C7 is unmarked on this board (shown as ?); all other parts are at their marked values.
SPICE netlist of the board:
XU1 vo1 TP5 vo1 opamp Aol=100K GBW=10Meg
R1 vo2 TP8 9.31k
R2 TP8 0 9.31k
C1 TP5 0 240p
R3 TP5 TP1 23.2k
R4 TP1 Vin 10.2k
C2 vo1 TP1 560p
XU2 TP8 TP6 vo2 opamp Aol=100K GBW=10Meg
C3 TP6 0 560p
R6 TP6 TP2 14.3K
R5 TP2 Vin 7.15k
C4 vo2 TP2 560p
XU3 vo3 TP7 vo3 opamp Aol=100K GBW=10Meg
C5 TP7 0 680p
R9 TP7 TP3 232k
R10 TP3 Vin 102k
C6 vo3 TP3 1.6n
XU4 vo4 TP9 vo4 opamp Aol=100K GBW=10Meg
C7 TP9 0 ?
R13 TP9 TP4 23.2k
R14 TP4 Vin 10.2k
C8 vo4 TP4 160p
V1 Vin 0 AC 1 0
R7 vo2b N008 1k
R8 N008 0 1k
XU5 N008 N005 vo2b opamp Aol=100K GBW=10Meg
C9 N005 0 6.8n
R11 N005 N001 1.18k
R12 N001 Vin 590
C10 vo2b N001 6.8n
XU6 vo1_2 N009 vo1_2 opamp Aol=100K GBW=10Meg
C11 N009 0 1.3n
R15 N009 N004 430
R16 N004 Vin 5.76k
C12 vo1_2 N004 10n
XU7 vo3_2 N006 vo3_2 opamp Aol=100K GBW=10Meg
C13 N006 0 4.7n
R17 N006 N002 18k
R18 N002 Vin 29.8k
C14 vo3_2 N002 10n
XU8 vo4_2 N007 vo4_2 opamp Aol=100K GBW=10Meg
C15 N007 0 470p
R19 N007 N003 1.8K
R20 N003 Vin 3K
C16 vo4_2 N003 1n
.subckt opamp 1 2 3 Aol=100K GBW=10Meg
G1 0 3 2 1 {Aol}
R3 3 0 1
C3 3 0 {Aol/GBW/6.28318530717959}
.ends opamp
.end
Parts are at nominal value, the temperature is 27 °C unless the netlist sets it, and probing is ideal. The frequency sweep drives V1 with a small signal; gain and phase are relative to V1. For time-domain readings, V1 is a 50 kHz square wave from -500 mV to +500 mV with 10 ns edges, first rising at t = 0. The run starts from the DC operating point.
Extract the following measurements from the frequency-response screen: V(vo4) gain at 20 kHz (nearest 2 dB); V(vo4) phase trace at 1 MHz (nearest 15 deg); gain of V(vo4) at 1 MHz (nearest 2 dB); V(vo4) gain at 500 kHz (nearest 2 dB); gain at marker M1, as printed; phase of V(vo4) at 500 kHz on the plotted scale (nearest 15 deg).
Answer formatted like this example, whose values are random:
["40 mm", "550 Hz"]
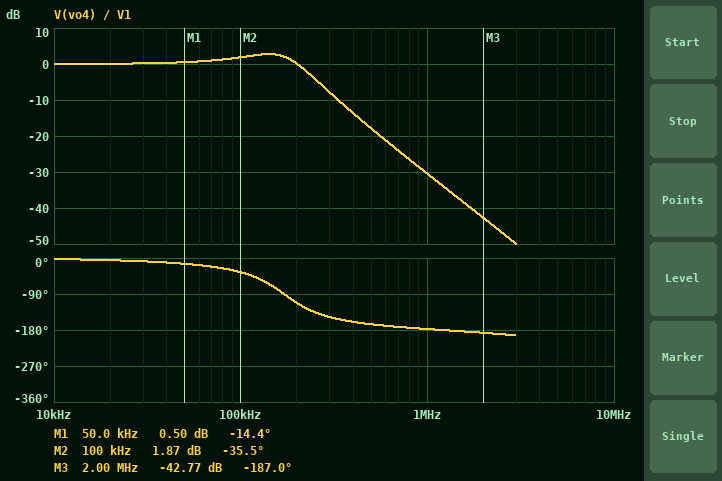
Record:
["0 dB", "-180 deg", "-30 dB", "-18 dB", "0.50 dB", "-165 deg"]
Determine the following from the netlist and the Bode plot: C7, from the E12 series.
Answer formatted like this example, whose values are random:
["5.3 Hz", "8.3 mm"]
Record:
["22 pF"]
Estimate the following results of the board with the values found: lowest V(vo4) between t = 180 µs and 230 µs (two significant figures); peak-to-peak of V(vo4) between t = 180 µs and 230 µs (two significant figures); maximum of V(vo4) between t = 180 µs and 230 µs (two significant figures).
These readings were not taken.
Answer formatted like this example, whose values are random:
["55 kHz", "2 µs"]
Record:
["-760 mV", "1.5 V", "760 mV"]
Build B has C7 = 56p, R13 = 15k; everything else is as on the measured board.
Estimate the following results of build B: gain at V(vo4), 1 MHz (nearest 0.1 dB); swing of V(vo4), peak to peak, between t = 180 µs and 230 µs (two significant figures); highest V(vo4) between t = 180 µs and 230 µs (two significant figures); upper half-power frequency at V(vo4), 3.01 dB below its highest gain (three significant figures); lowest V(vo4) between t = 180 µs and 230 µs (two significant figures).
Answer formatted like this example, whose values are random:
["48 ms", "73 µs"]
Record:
["-34.8 dB", "1.2 V", "600 mV", "150 kHz", "-600 mV"]
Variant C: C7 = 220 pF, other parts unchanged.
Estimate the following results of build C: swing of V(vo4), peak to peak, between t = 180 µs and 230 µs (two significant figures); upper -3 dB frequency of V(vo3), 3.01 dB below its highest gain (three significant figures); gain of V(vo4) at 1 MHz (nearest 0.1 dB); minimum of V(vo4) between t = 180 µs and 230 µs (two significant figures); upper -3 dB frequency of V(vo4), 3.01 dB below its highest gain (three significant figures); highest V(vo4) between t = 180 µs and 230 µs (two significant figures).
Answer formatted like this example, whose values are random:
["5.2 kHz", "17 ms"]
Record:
["600 mV", "991 Hz", "-50.5 dB", "-300 mV", "25.5 kHz", "300 mV"]
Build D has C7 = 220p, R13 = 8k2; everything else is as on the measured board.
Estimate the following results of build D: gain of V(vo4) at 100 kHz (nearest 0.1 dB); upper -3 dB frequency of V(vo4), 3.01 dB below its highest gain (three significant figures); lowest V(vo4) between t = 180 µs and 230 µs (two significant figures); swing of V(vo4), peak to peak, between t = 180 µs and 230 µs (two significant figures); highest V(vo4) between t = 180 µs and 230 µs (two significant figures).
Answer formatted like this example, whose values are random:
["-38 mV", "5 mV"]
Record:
["-8.1 dB", "47.5 kHz", "-450 mV", "890 mV", "450 mV"]
